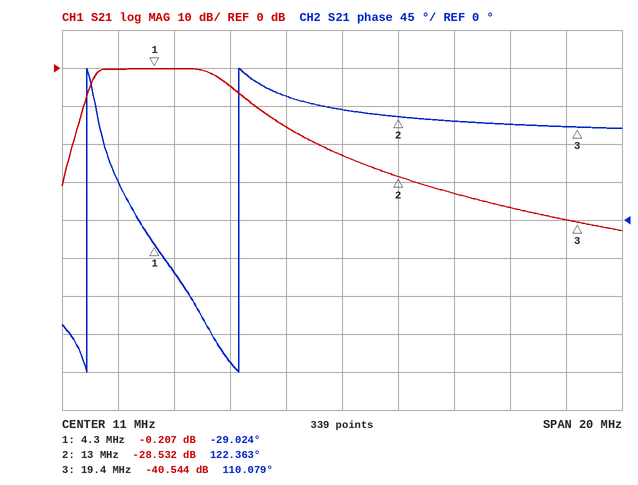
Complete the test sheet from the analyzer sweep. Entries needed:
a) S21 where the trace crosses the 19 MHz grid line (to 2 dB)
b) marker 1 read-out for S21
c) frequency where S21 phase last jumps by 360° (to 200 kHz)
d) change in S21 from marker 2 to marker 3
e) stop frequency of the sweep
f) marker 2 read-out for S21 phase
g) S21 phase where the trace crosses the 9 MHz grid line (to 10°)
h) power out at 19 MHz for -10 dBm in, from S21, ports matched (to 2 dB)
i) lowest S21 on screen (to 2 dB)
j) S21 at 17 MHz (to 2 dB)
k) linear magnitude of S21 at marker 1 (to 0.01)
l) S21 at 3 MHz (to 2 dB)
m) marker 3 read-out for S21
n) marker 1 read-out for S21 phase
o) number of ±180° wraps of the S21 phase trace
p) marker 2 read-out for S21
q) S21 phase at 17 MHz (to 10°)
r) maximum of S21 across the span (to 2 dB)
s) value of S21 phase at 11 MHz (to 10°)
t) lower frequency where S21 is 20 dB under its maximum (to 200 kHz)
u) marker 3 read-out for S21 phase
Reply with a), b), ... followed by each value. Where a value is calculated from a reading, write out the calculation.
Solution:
a) -40 dB
b) -0.207 dB
c) 7.4 MHz
d) -40.544 − (-28.532) = -12.012 dB
e) 21 MHz
f) 122.363°
g) 150°
h) -10 dBm + (-40 dB) = -50 dBm
i) -42 dB
j) -36 dB
k) 10^(-0.207/20) ≈ 0.98
l) 0 dB
m) -40.544 dB
n) -29.024°
o) 2
p) -28.532 dB
q) 110°
r) 0 dB
s) 130°
t) 1.4 MHz
u) 110.079°
